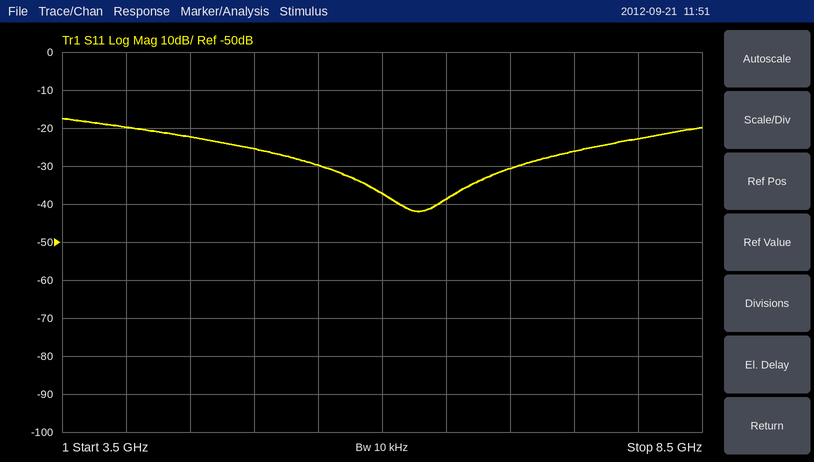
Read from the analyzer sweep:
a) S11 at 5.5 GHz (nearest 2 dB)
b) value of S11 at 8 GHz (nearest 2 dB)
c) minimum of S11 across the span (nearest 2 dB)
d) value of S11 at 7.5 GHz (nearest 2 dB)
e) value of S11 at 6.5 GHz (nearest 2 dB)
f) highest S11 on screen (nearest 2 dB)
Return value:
-30 dB
-22 dB
-42 dB
-26 dB
-38 dB
-18 dB
